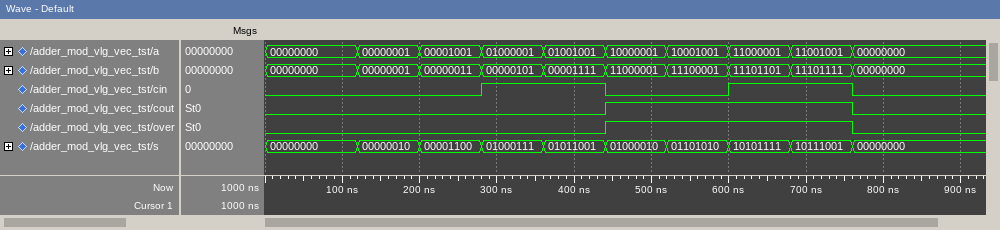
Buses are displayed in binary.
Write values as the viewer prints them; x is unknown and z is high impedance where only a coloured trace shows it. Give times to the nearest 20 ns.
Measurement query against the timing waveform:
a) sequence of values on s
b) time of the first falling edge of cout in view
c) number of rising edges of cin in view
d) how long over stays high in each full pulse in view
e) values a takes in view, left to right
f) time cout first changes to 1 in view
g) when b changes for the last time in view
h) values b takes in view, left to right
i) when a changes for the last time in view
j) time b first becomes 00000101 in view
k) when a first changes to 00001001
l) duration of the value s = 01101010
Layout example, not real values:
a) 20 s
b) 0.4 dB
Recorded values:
a) 00000000, 00000010, 00001100, 01000111, 01011001, 01000010, 01101010, 10101111, 10111001, 00000000
b) 760 ns
c) 2
d) 320 ns
e) 00000000, 00000001, 00001001, 01000001, 01001001, 10000001, 10001001, 11000001, 11001001, 00000000
f) 440 ns
g) 760 ns
h) 00000000, 00000001, 00000011, 00000101, 00001111, 11000001, 11100001, 11101101, 11101111, 00000000
i) 760 ns
j) 280 ns
k) 200 ns
l) 80 ns
